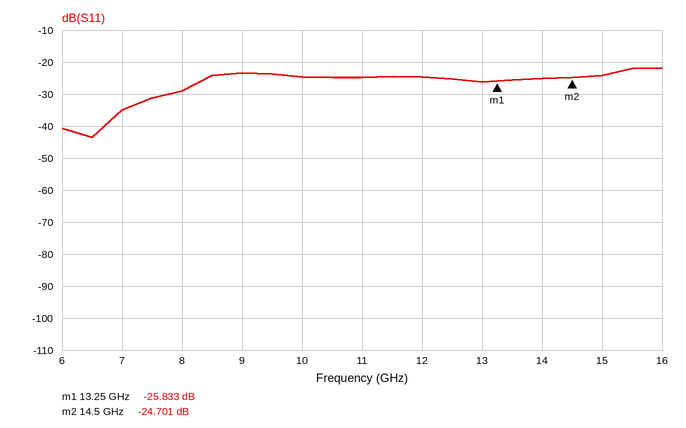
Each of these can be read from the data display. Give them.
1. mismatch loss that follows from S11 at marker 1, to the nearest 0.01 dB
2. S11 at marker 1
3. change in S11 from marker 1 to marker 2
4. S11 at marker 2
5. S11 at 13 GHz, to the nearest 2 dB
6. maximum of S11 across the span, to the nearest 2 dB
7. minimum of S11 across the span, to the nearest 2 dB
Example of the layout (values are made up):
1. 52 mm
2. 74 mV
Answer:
1. 0.01 dB
2. -25.833 dB
3. 1.132 dB
4. -24.701 dB
5. -26 dB
6. -22 dB
7. -44 dB
